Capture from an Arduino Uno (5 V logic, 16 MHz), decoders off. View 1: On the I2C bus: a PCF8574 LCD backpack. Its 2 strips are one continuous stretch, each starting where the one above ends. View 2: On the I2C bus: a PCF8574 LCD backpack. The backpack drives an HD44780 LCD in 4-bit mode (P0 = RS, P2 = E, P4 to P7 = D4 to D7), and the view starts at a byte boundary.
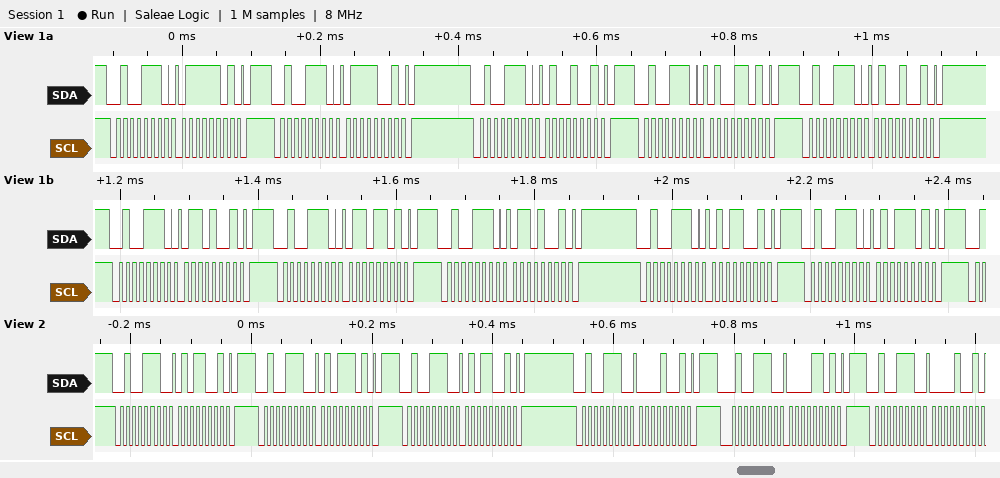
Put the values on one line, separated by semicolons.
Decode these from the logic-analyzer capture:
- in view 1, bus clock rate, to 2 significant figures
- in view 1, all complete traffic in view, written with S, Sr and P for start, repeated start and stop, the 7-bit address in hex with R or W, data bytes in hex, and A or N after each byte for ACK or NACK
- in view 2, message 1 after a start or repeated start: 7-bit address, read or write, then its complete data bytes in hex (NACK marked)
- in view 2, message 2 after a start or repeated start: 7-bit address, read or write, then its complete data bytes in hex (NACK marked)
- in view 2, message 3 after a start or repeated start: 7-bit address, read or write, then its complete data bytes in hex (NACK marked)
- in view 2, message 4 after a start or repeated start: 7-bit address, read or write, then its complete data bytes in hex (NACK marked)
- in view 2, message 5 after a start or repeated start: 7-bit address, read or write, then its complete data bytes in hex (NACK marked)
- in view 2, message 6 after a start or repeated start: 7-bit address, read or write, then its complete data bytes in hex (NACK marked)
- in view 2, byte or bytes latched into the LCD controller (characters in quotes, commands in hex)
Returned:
100 kHz; S 27W A 7D A P S 27W A 79 A P S 27W A 49 A P S 27W A 4D A P S 27W A 49 A P S 27W A 69 A P S 27W A 6D A P S 27W A 69 A P S 27W A 59 A P S 27W A 5D A P; 0x27 write: 59; 0x27 write: 5D; 0x27 write: 59; 0x27 write: 09; 0x27 write: 0D; 0x27 write: 09; 'P'
